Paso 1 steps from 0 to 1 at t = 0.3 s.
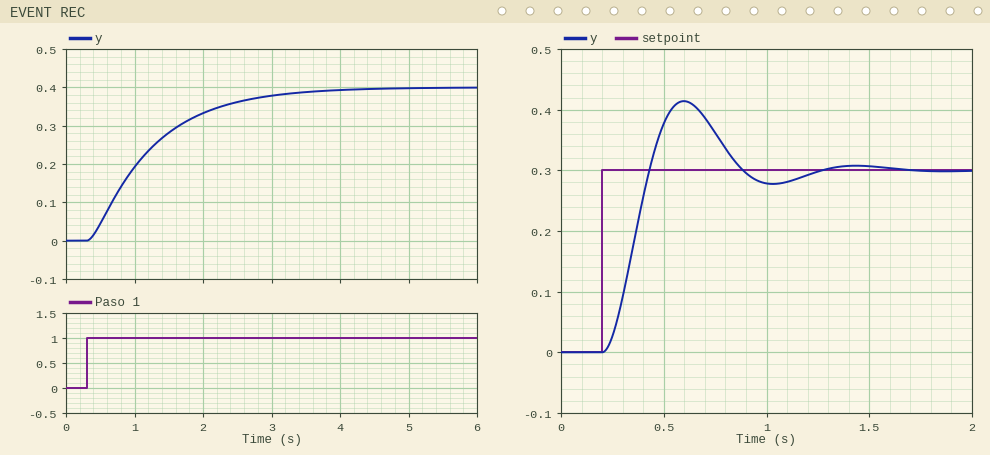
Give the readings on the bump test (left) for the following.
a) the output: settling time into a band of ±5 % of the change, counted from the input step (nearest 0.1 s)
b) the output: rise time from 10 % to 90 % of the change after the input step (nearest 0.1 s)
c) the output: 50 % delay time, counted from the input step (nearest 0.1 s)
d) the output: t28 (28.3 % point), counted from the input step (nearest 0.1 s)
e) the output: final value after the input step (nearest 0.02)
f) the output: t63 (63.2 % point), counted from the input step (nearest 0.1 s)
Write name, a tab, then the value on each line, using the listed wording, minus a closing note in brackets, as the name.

the output: settling time into a band of ±5 % of the change, counted from the input step	2.8 s
the output: rise time from 10 % to 90 % of the change after the input step	2.0 s
the output: 50 % delay time, counted from the input step	0.7 s
the output: t28 (28.3 % point), counted from the input step	0.4 s
the output: final value after the input step	0.40
the output: t63 (63.2 % point), counted from the input step	1.0 s
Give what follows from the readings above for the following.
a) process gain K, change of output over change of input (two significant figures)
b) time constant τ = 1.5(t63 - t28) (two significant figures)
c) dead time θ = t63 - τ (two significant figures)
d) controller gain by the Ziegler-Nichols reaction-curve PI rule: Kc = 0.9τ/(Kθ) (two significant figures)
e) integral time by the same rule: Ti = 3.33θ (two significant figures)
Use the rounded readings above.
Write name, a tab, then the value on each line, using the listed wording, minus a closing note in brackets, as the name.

process gain K, change of output over change of input	0.40
time constant τ = 1.5(t63 - t28)	0.90 s
dead time θ = t63 - τ	0.10 s
controller gain by the Ziegler-Nichols reaction-curve PI rule: Kc = 0.9τ/(Kθ)	20
integral time by the same rule: Ti = 3.33θ	0.33 s
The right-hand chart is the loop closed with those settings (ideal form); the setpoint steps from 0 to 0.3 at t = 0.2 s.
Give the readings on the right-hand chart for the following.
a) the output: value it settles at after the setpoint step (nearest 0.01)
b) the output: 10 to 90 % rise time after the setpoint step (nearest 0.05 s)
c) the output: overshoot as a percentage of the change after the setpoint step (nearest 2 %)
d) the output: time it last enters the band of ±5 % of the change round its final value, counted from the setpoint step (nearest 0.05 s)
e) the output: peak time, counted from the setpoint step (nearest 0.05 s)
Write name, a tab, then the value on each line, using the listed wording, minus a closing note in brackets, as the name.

the output: value it settles at after the setpoint step	0.30
the output: 10 to 90 % rise time after the setpoint step	0.15 s
the output: overshoot as a percentage of the change after the setpoint step	38 %
the output: time it last enters the band of ±5 % of the change round its final value, counted from the setpoint step	0.95 s
the output: peak time, counted from the setpoint step	0.40 s
